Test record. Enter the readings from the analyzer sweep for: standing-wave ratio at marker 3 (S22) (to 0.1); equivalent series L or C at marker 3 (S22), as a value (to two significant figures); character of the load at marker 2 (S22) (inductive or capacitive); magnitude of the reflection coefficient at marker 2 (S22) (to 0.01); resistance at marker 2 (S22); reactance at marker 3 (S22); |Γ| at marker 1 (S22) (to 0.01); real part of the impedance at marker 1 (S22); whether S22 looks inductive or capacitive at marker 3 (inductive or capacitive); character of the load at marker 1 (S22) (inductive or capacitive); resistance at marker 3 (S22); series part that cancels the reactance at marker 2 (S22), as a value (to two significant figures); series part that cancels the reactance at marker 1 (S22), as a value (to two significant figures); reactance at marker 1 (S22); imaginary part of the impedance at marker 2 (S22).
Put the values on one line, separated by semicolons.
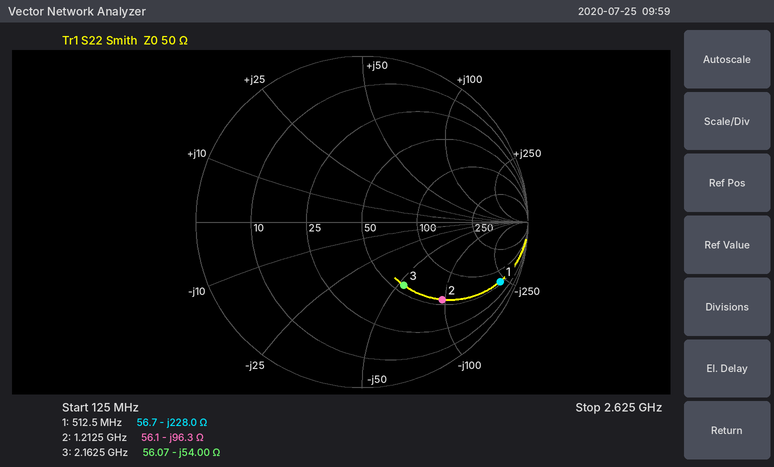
2.7; 1.4 pF; capacitive; 0.67; 56.1 Ω; -54.00 Ω; 0.91; 56.7 Ω; capacitive; capacitive; 56.07 Ω; 13 nH; 71 nH; -228.0 Ω; -96.3 Ω
